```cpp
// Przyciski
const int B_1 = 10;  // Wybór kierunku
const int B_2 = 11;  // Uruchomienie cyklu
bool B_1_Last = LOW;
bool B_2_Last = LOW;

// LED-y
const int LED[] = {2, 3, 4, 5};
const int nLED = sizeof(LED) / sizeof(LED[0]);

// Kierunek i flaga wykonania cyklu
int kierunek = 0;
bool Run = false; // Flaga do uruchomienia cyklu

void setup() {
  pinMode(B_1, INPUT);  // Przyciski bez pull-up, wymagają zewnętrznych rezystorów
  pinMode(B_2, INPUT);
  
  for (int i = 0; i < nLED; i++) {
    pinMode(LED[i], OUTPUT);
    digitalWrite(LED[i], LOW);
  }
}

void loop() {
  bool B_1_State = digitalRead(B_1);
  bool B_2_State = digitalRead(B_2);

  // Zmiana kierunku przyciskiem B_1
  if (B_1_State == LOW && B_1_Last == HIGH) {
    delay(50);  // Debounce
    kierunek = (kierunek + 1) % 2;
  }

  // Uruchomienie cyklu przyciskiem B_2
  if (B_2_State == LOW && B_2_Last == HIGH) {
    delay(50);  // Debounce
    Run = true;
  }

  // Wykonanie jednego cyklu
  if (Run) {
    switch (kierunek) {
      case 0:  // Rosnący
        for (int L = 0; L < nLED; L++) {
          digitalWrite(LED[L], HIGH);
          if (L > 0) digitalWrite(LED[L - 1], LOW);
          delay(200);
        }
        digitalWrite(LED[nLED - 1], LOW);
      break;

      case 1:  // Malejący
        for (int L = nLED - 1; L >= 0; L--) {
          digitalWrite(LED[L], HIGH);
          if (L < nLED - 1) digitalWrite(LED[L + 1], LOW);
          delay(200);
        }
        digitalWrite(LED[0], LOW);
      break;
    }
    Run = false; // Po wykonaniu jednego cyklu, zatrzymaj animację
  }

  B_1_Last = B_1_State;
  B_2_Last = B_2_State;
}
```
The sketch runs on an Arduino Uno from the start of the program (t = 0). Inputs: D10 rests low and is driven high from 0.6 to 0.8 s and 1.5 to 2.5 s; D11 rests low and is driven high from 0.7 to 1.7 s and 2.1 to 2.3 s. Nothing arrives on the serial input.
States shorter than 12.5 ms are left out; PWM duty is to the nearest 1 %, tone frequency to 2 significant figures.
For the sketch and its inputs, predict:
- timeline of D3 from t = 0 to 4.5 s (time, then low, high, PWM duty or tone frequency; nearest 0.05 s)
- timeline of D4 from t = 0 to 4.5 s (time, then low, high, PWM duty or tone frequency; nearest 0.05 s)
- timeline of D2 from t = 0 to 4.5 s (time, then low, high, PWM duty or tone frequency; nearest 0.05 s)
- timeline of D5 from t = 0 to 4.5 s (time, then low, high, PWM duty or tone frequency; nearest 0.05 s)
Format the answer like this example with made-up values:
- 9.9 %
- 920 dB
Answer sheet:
- 0 s low; 2.15 s high; 2.35 s low
- 0 s low; 1.95 s high; 2.15 s low
- 0 s low; 2.35 s high; 2.55 s low
- 0 s low; 1.75 s high; 1.95 s low
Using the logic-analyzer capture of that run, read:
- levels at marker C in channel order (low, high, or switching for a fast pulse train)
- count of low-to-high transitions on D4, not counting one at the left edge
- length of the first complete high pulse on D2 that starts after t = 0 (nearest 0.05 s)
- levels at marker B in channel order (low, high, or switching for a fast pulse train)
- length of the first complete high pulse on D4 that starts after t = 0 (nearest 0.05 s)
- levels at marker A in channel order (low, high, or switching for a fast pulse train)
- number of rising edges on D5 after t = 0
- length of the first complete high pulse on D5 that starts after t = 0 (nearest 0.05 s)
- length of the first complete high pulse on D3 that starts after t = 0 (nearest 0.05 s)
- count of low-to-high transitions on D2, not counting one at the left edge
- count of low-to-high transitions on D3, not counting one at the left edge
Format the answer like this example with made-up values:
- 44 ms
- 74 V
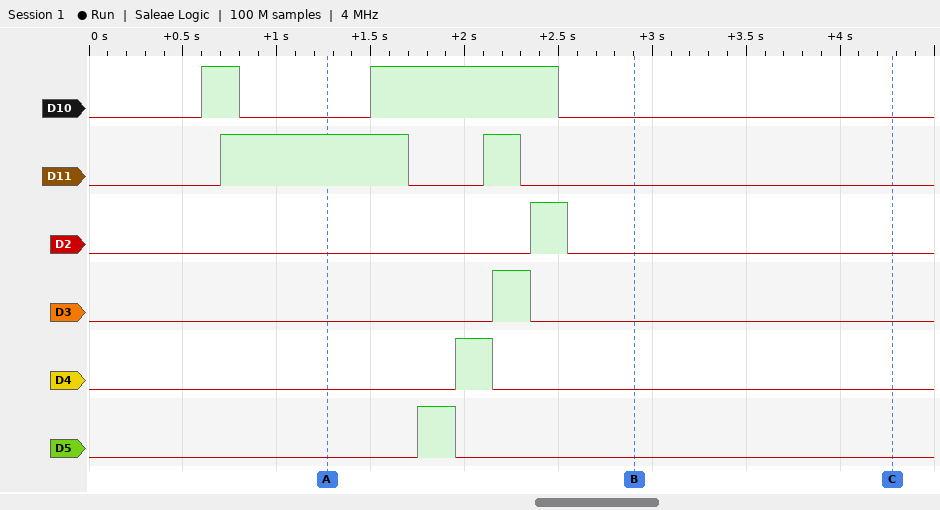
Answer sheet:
- D10 low, D11 low, D2 low, D3 low, D4 low, D5 low
- 1
- 0.20 s
- D10 low, D11 low, D2 low, D3 low, D4 low, D5 low
- 0.20 s
- D10 low, D11 high, D2 low, D3 low, D4 low, D5 low
- 1
- 0.20 s
- 0.20 s
- 1
- 1
